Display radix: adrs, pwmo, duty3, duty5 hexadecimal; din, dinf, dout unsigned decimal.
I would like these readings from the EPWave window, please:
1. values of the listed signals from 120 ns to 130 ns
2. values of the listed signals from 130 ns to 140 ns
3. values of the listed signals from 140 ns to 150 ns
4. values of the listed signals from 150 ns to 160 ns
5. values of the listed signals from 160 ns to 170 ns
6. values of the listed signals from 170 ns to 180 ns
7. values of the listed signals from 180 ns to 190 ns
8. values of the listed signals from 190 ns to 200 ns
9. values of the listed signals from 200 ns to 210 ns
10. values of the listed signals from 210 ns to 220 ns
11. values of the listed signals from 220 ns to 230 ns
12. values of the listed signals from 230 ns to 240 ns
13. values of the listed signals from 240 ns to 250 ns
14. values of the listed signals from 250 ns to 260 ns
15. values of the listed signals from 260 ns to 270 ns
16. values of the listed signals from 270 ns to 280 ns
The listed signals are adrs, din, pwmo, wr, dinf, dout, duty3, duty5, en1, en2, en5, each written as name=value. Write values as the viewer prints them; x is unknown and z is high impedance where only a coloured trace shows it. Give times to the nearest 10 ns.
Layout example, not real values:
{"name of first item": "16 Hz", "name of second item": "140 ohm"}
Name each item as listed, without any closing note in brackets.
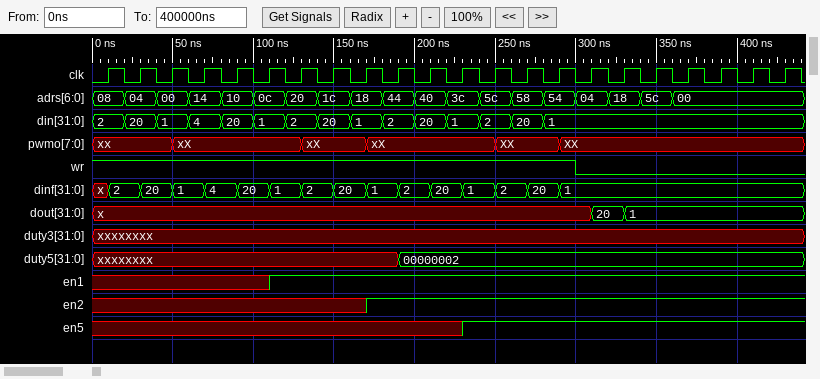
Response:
{"values of the listed signals from 120 ns to 130 ns": "adrs=20, din=2, pwmo=xX, wr=1, dinf=1, dout=x, duty3=xxxxxxxx, duty5=xxxxxxxx, en1=1, en2=x, en5=x", "values of the listed signals from 130 ns to 140 ns": "adrs=20, din=2, pwmo=xX, wr=1, dinf=2, dout=x, duty3=xxxxxxxx, duty5=xxxxxxxx, en1=1, en2=x, en5=x", "values of the listed signals from 140 ns to 150 ns": "adrs=1c, din=20, pwmo=xX, wr=1, dinf=2, dout=x, duty3=xxxxxxxx, duty5=xxxxxxxx, en1=1, en2=x, en5=x", "values of the listed signals from 150 ns to 160 ns": "adrs=1c, din=20, pwmo=xX, wr=1, dinf=20, dout=x, duty3=xxxxxxxx, duty5=xxxxxxxx, en1=1, en2=x, en5=x", "values of the listed signals from 160 ns to 170 ns": "adrs=18, din=1, pwmo=xX, wr=1, dinf=20, dout=x, duty3=xxxxxxxx, duty5=xxxxxxxx, en1=1, en2=x, en5=x", "values of the listed signals from 170 ns to 180 ns": "adrs=18, din=1, pwmo=xX, wr=1, dinf=1, dout=x, duty3=xxxxxxxx, duty5=xxxxxxxx, en1=1, en2=1, en5=x", "values of the listed signals from 180 ns to 190 ns": "adrs=44, din=2, pwmo=xX, wr=1, dinf=1, dout=x, duty3=xxxxxxxx, duty5=xxxxxxxx, en1=1, en2=1, en5=x", "values of the listed signals from 190 ns to 200 ns": "adrs=44, din=2, pwmo=xX, wr=1, dinf=2, dout=x, duty3=xxxxxxxx, duty5=00000002, en1=1, en2=1, en5=x", "values of the listed signals from 200 ns to 210 ns": "adrs=40, din=20, pwmo=xX, wr=1, dinf=2, dout=x, duty3=xxxxxxxx, duty5=00000002, en1=1, en2=1, en5=x", "values of the listed signals from 210 ns to 220 ns": "adrs=40, din=20, pwmo=xX, wr=1, dinf=20, dout=x, duty3=xxxxxxxx, duty5=00000002, en1=1, en2=1, en5=x", "values of the listed signals from 220 ns to 230 ns": "adrs=3c, din=1, pwmo=xX, wr=1, dinf=20, dout=x, duty3=xxxxxxxx, duty5=00000002, en1=1, en2=1, en5=x", "values of the listed signals from 230 ns to 240 ns": "adrs=3c, din=1, pwmo=xX, wr=1, dinf=1, dout=x, duty3=xxxxxxxx, duty5=00000002, en1=1, en2=1, en5=1", "values of the listed signals from 240 ns to 250 ns": "adrs=5c, din=2, pwmo=xX, wr=1, dinf=1, dout=x, duty3=xxxxxxxx, duty5=00000002, en1=1, en2=1, en5=1", "values of the listed signals from 250 ns to 260 ns": "adrs=5c, din=2, pwmo=XX, wr=1, dinf=2, dout=x, duty3=xxxxxxxx, duty5=00000002, en1=1, en2=1, en5=1", "values of the listed signals from 260 ns to 270 ns": "adrs=58, din=20, pwmo=XX, wr=1, dinf=2, dout=x, duty3=xxxxxxxx, duty5=00000002, en1=1, en2=1, en5=1", "values of the listed signals from 270 ns to 280 ns": "adrs=58, din=20, pwmo=XX, wr=1, dinf=20, dout=x, duty3=xxxxxxxx, duty5=00000002, en1=1, en2=1, en5=1"}
